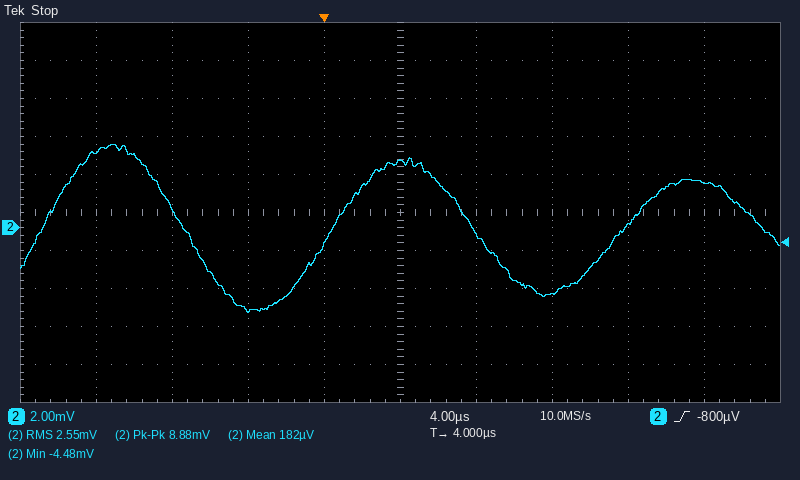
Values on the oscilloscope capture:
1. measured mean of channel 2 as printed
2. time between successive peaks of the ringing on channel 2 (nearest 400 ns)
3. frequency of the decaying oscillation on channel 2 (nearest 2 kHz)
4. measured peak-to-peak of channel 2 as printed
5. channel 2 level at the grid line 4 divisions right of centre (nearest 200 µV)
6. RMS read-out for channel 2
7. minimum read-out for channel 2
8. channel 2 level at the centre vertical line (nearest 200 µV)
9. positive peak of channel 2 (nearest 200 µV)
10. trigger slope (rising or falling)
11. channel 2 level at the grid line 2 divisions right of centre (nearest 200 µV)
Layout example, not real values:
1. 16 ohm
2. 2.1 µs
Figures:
1. 182 µV
2. 15.2 µs
3. 66 kHz
4. 8.88 mV
5. 2.4 mV
6. 2.55 mV
7. -4.48 mV
8. 3.4 mV
9. 4.4 mV
10. rising
11. -3.4 mV
